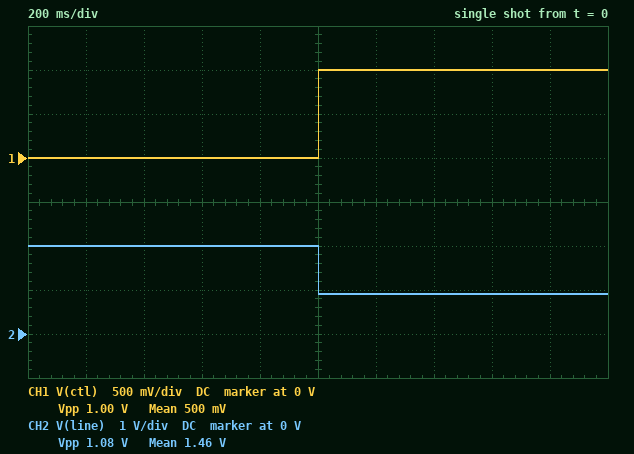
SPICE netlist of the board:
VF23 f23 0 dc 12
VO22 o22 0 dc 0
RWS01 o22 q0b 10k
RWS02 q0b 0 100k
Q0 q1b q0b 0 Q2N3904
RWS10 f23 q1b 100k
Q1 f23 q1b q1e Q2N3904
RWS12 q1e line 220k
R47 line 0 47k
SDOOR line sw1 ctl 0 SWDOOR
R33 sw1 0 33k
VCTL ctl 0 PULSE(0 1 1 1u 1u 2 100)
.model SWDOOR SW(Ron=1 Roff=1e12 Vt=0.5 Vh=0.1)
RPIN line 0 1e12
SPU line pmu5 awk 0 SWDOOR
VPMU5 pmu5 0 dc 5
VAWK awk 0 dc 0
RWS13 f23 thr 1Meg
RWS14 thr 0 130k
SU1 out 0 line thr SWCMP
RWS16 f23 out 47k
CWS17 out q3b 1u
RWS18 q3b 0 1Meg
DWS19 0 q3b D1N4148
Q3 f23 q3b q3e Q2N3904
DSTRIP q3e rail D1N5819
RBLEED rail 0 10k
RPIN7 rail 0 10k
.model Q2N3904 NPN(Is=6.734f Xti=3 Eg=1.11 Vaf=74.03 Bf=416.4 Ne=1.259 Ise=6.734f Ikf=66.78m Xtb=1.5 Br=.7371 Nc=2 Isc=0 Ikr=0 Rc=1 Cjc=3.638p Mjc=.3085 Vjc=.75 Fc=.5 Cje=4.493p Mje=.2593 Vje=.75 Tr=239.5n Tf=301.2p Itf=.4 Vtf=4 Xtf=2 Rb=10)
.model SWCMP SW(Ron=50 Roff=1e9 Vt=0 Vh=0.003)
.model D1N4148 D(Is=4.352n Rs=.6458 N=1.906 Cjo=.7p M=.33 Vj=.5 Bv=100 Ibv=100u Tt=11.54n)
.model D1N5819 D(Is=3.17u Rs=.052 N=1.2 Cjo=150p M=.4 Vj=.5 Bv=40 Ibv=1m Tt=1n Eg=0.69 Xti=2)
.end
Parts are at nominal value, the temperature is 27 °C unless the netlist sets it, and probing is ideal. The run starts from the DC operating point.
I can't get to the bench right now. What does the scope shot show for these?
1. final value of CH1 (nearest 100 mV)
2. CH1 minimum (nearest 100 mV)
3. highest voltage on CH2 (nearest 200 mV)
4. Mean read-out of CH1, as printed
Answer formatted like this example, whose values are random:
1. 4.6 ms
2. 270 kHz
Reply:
1. 1.0 V
2. 0 V
3. 2.0 V
4. 500 mV
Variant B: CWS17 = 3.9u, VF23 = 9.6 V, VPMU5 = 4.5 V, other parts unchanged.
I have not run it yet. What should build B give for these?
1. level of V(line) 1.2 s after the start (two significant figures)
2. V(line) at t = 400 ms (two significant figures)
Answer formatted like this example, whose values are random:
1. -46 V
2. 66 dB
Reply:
1. 730 mV
2. 1.6 V
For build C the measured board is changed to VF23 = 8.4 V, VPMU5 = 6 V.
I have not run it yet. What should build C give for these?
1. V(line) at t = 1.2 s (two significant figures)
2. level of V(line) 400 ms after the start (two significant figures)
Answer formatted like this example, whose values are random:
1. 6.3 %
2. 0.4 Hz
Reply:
1. 630 mV
2. 1.4 V
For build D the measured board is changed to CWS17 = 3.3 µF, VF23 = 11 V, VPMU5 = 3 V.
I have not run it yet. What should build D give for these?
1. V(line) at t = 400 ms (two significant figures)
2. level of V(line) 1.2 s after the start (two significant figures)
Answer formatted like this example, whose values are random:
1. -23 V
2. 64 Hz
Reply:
1. 1.8 V
2. 840 mV
